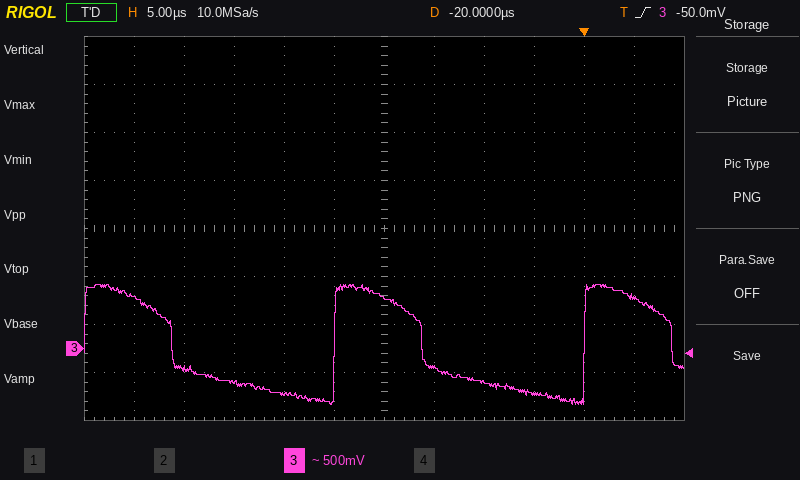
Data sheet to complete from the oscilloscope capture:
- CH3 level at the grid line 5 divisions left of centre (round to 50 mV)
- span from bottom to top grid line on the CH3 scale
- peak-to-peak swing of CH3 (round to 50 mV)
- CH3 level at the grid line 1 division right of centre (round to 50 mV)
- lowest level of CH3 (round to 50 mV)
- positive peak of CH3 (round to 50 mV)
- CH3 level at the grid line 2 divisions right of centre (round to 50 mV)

550 mV
4 V
1.25 V
-200 mV
-600 mV
650 mV
-350 mV
